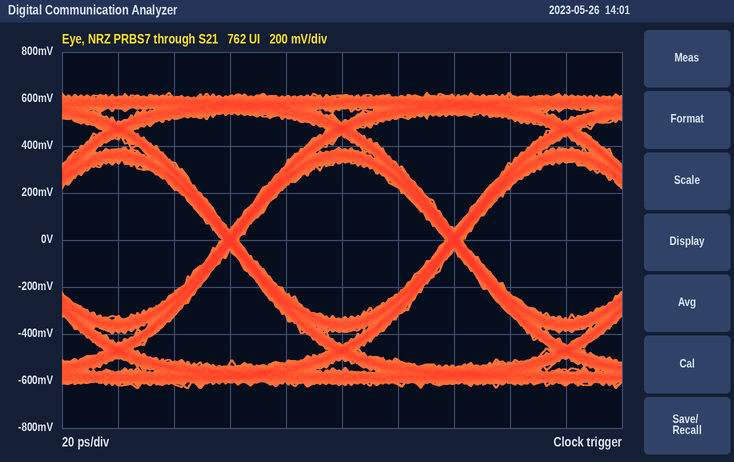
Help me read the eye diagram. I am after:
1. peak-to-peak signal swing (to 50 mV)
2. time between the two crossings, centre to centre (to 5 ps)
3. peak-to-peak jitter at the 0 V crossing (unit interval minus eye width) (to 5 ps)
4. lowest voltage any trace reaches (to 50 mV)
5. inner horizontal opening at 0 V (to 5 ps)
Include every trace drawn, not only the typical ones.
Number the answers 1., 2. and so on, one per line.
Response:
1. 1.25 V
2. 80 ps
3. 5 ps
4. -650 mV
5. 75 ps
